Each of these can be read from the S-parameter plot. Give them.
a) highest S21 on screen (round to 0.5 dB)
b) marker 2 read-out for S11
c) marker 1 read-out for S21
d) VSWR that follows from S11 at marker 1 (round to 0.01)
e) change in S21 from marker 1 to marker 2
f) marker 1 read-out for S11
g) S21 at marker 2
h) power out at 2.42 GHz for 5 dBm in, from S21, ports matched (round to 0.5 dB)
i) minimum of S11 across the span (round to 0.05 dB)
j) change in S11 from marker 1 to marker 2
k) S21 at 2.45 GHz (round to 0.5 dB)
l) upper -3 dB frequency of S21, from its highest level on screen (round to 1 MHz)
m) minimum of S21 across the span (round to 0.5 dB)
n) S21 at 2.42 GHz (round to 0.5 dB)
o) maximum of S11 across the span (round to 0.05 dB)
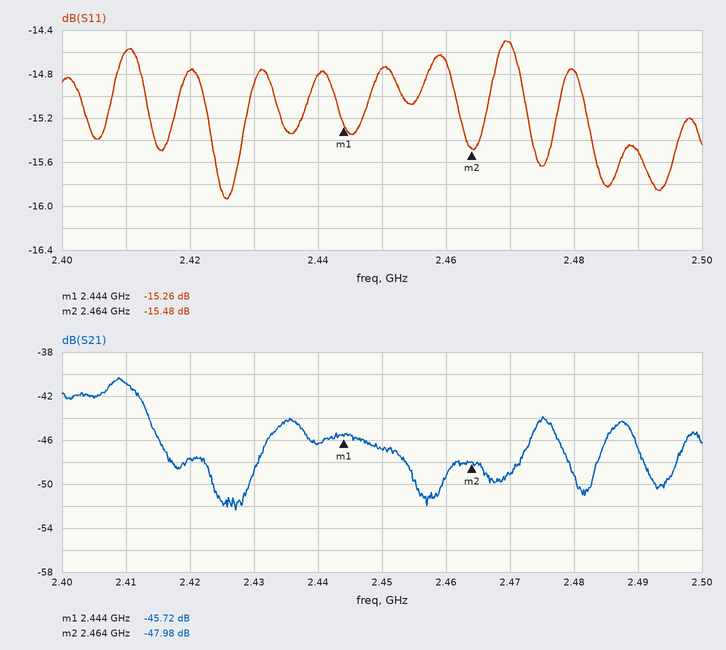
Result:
-40.5 dB
-15.48 dB
-45.72 dB
1.42
-2.26 dB
-15.26 dB
-47.98 dB
-42.5 dBm
-15.95 dB
-0.22 dB
-47.0 dB
2.413 GHz
-52.5 dB
-47.5 dB
-14.50 dB
